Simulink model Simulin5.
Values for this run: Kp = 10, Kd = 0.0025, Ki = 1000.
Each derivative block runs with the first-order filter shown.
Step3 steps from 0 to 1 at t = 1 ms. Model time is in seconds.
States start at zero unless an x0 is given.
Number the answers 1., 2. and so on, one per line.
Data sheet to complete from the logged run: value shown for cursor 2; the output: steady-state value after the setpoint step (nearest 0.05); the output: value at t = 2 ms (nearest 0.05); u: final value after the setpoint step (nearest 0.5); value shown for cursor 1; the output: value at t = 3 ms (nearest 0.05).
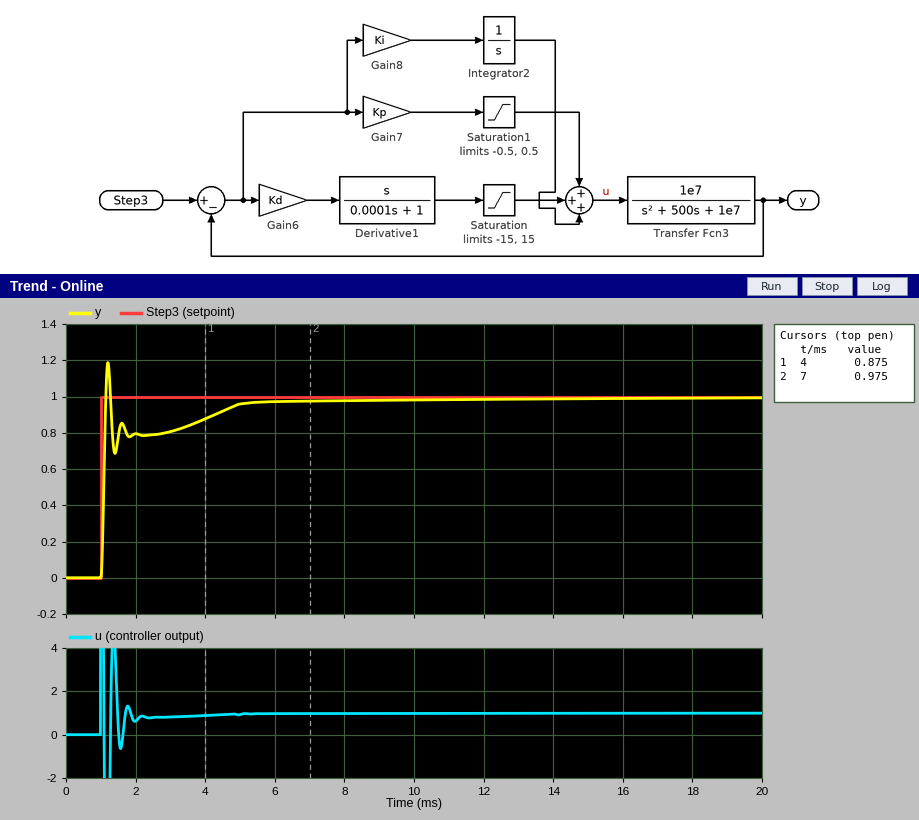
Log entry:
1. 0.975
2. 1.00
3. 0.80
4. 1.0
5. 0.875
6. 0.80
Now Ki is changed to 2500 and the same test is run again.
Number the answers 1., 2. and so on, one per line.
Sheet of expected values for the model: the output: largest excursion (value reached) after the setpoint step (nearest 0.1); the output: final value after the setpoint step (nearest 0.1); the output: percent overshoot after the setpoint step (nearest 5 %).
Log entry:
1. 1.2
2. 1.0
3. 20 %
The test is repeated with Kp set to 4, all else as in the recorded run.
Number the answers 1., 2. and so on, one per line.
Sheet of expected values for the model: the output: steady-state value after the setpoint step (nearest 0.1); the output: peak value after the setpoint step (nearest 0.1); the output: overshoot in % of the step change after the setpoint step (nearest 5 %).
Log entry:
1. 1.0
2. 1.2
3. 20 %
